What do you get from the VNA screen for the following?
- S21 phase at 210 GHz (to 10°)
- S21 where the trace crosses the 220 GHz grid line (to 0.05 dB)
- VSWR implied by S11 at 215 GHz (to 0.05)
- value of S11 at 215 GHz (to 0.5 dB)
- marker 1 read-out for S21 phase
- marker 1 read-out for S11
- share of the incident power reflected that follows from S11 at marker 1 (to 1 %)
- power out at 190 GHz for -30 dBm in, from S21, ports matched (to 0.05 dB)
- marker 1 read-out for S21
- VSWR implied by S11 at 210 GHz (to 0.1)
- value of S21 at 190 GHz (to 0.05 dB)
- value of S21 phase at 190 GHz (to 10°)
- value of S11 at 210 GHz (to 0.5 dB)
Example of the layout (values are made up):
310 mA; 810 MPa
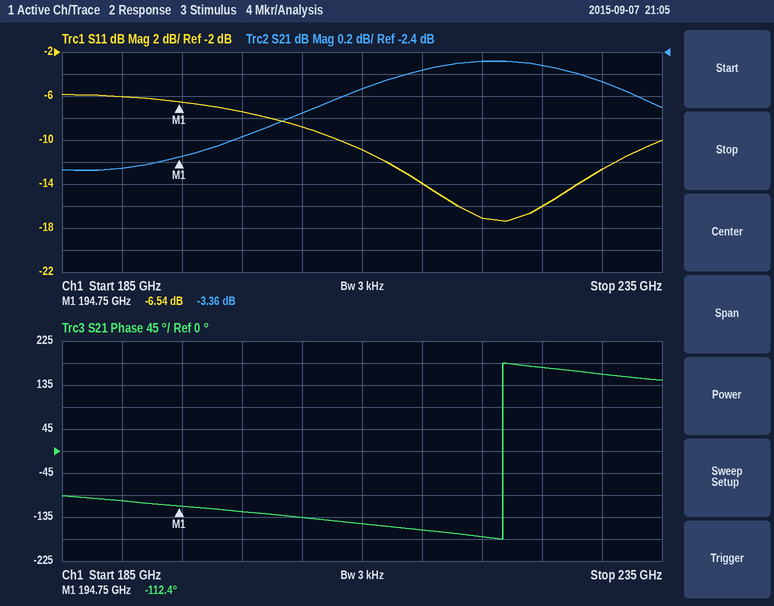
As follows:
-150°; -2.50 dB; 1.50; -14.0 dB; -112.4°; -6.54 dB; 22 %; -33.45 dBm; -3.36 dB; 1.8; -3.45 dB; -100°; -11.0 dB
